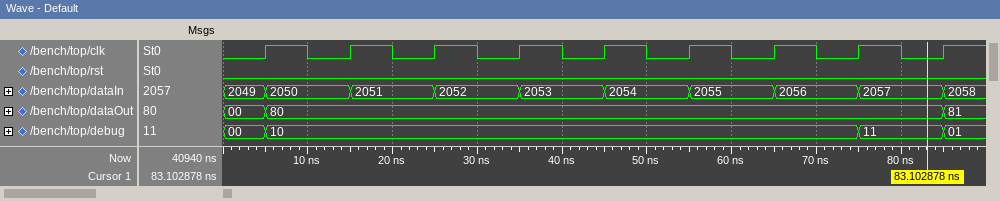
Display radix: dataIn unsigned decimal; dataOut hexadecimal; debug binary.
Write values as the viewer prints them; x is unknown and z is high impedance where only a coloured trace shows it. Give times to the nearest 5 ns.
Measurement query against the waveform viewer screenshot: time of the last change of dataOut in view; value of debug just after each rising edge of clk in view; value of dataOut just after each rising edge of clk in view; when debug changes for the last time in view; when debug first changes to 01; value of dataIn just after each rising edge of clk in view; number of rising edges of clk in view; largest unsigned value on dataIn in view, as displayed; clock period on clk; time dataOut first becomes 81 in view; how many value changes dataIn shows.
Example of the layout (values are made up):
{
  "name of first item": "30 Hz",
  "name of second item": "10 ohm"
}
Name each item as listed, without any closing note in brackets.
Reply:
{
  "time of the last change of dataOut in view": "85 ns",
  "value of debug just after each rising edge of clk in view": "10, 10, 10, 10, 10, 10, 10, 11, 01",
  "value of dataOut just after each rising edge of clk in view": "80, 80, 80, 80, 80, 80, 80, 80, 81",
  "when debug changes for the last time in view": "85 ns",
  "when debug first changes to 01": "85 ns",
  "value of dataIn just after each rising edge of clk in view": "2050, 2051, 2052, 2053, 2054, 2055, 2056, 2057, 2058",
  "number of rising edges of clk in view": "9",
  "largest unsigned value on dataIn in view, as displayed": "2058",
  "clock period on clk": "10 ns",
  "time dataOut first becomes 81 in view": "85 ns",
  "how many value changes dataIn shows": "9"
}
